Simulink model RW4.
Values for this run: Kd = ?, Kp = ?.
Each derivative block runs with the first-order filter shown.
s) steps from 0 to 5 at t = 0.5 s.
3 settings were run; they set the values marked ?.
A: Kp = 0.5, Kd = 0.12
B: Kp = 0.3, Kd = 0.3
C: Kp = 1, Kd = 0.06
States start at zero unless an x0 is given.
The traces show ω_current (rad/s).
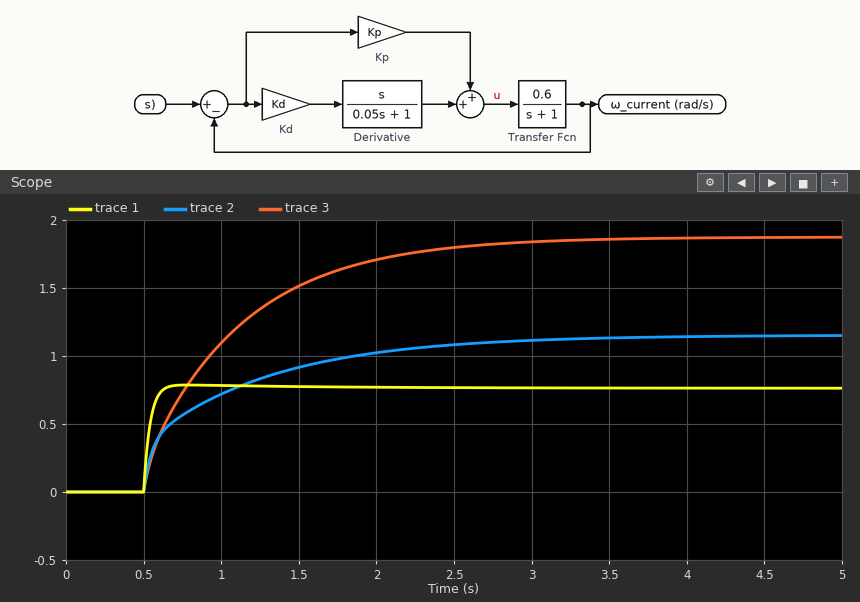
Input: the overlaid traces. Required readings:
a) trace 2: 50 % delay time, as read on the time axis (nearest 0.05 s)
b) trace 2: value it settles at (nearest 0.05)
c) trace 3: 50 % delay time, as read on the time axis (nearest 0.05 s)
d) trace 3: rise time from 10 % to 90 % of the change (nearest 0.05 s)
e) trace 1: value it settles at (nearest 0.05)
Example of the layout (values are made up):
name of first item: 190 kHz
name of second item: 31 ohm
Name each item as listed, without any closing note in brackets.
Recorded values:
trace 2: 50 % delay time, as read on the time axis: 0.75 s
trace 2: value it settles at: 1.15
trace 3: 50 % delay time, as read on the time axis: 0.90 s
trace 3: rise time from 10 % to 90 % of the change: 1.40 s
trace 1: value it settles at: 0.75
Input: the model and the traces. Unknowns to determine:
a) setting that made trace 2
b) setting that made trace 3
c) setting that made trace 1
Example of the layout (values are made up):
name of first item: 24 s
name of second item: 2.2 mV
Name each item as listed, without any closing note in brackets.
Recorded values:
setting that made trace 2: A
setting that made trace 3: C
setting that made trace 1: B
